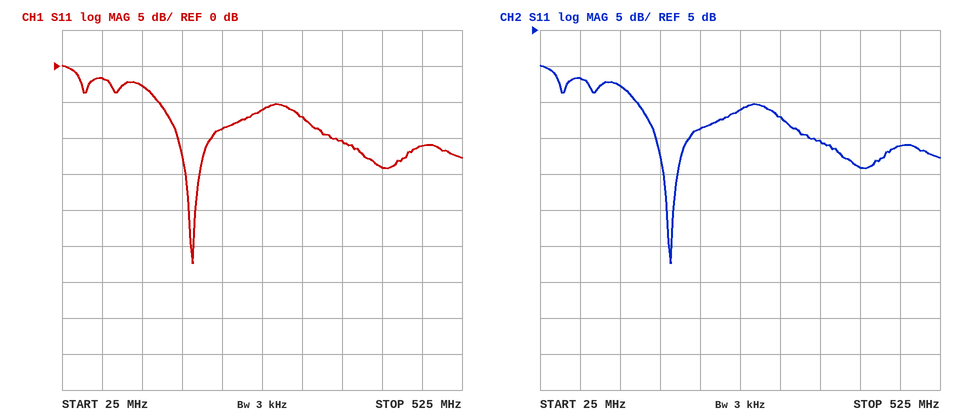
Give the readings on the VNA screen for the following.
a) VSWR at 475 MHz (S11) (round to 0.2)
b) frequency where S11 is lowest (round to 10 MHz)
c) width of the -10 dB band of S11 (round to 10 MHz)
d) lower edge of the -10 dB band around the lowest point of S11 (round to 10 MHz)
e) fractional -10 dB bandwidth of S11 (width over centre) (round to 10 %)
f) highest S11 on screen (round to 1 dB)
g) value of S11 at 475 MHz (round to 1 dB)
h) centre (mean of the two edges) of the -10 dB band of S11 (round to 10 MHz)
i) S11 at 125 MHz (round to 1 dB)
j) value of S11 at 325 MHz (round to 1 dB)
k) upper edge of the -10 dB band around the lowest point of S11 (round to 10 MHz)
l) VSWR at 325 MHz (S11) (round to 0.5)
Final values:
1.8
190 MHz
40 MHz
170 MHz
20 %
0 dB
-11 dB
190 MHz
-3 dB
-7 dB
210 MHz
2.5
